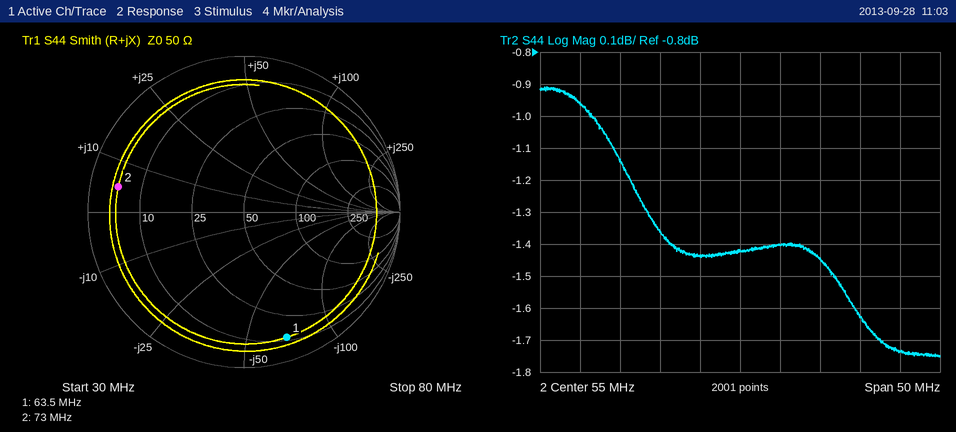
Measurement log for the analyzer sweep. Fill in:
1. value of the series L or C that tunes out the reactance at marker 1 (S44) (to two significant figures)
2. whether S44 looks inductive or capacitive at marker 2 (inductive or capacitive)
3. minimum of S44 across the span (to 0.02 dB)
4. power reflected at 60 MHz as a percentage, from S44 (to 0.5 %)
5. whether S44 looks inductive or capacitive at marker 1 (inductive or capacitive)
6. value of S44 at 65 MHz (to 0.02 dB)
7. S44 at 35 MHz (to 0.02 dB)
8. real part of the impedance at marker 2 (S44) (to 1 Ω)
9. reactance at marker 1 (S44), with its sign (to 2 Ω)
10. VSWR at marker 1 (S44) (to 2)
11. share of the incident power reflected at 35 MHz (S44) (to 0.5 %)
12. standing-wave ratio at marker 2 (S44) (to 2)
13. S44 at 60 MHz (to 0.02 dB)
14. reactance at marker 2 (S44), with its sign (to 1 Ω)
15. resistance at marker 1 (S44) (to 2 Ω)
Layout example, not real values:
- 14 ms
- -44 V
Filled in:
- 170 nH
- inductive
- -1.76 dB
- 72.5 %
- capacitive
- -1.44 dB
- -0.96 dB
- 5 Ω
- -68 Ω
- 12
- 80.0 %
- 10
- -1.40 dB
- +5 Ω
- 12 Ω
